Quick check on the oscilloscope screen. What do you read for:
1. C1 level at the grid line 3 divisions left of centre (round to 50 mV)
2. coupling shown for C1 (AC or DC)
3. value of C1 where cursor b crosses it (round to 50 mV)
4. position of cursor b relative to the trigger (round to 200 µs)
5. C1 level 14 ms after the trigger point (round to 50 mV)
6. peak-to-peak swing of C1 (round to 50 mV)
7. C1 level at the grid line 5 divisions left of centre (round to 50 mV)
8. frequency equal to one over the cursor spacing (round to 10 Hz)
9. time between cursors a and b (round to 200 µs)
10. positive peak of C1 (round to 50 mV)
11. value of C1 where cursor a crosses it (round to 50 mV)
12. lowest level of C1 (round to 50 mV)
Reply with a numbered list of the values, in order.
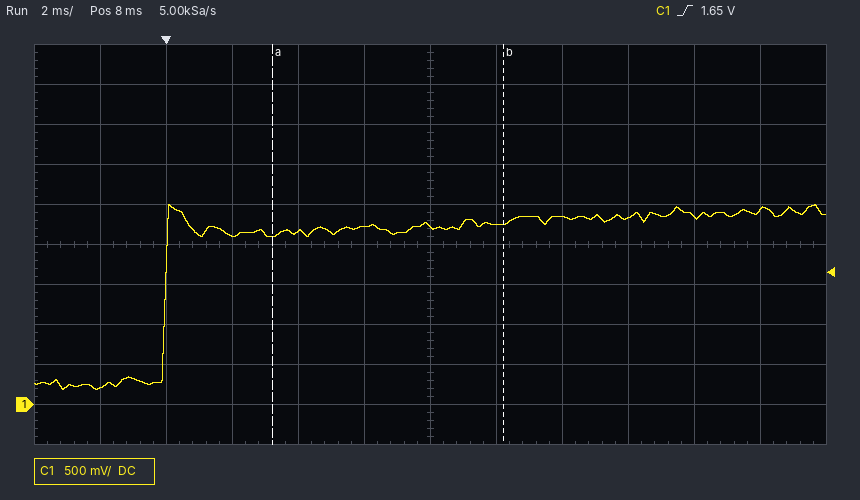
1. 2.10 V
2. DC
3. 2.25 V
4. +10.2 ms
5. 2.35 V
6. 2.30 V
7. 200 mV
8. 140 Hz
9. 7.0 ms
10. 2.50 V
11. 2.10 V
12. 200 mV
